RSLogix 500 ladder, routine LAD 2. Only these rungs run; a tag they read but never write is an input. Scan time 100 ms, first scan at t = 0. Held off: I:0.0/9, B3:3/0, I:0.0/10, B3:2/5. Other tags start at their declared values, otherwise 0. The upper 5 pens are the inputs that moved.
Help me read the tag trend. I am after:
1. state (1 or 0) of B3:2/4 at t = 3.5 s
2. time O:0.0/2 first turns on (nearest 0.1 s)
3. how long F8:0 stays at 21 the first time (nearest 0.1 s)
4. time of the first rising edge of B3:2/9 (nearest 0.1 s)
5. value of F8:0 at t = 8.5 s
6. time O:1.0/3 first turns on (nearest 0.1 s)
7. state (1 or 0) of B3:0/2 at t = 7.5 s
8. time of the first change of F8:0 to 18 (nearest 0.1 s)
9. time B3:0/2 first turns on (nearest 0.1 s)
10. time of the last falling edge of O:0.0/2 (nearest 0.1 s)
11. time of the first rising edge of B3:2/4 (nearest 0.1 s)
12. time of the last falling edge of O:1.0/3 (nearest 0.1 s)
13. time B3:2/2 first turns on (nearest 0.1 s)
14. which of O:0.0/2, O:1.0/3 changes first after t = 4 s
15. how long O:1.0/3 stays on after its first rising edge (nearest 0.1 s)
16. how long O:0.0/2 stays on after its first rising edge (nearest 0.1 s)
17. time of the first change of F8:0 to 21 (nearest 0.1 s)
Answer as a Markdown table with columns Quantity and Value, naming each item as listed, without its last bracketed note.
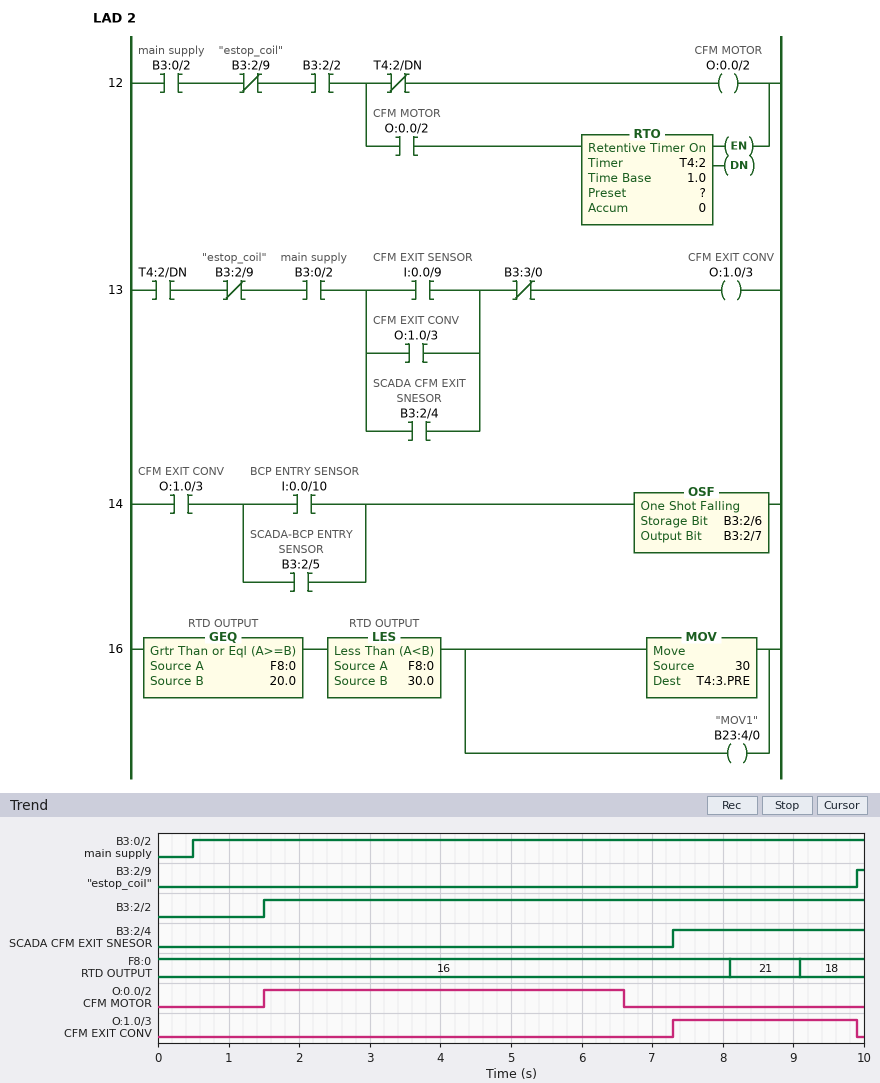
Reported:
| Quantity | Value |
|---|---|
| state (1 or 0) of B3:2/4 at t = 3.5 s | 0 |
| time O:0.0/2 first turns on | 1.5 s |
| how long F8:0 stays at 21 the first time | 1.0 s |
| time of the first rising edge of B3:2/9 | 9.9 s |
| value of F8:0 at t = 8.5 s | 21 |
| time O:1.0/3 first turns on | 7.3 s |
| state (1 or 0) of B3:0/2 at t = 7.5 s | 1 |
| time of the first change of F8:0 to 18 | 9.1 s |
| time B3:0/2 first turns on | 0.5 s |
| time of the last falling edge of O:0.0/2 | 6.6 s |
| time of the first rising edge of B3:2/4 | 7.3 s |
| time of the last falling edge of O:1.0/3 | 9.9 s |
| time B3:2/2 first turns on | 1.5 s |
| which of O:0.0/2, O:1.0/3 changes first after t = 4 s | O:0.0/2 |
| how long O:1.0/3 stays on after its first rising edge | 2.6 s |
| how long O:0.0/2 stays on after its first rising edge | 5.1 s |
| time of the first change of F8:0 to 21 | 8.1 s |
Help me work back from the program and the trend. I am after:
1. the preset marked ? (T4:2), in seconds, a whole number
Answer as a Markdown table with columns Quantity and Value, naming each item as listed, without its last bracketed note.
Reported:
| Quantity | Value |
|---|---|
| the preset marked ? (T4:2), in seconds, a whole number | 5 s |
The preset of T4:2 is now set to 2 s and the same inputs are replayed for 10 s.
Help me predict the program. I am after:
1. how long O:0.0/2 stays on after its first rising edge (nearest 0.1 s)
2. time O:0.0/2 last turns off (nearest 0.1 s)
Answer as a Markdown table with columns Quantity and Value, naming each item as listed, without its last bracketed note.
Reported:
| Quantity | Value |
|---|---|
| how long O:0.0/2 stays on after its first rising edge | 2.1 s |
| time O:0.0/2 last turns off | 3.6 s |
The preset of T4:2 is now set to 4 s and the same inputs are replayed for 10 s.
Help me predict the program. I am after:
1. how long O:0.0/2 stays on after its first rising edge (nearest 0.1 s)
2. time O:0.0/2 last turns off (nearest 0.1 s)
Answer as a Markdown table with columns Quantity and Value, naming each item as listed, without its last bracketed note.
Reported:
| Quantity | Value |
|---|---|
| how long O:0.0/2 stays on after its first rising edge | 4.1 s |
| time O:0.0/2 last turns off | 5.6 s |
